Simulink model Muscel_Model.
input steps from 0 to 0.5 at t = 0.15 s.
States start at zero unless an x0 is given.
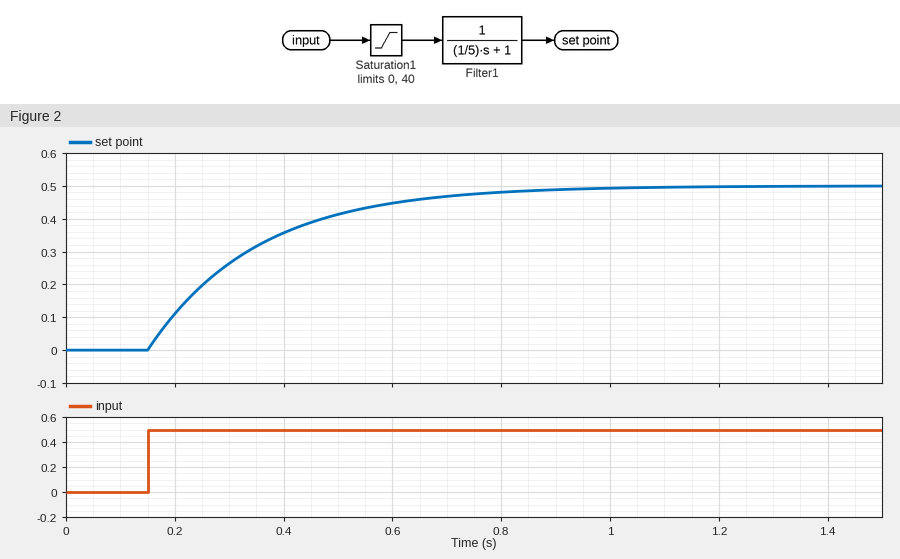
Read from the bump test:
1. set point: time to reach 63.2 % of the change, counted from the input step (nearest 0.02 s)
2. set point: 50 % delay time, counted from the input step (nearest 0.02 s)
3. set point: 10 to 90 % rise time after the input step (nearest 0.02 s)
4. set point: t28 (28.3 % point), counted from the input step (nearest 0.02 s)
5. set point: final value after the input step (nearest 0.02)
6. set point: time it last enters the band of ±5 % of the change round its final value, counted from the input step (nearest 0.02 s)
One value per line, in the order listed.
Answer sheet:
0.20 s
0.14 s
0.44 s
0.06 s
0.50
0.60 s
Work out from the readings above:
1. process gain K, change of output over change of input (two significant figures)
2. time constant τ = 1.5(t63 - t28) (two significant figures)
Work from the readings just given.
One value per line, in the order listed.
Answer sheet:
1.0
0.21 s
